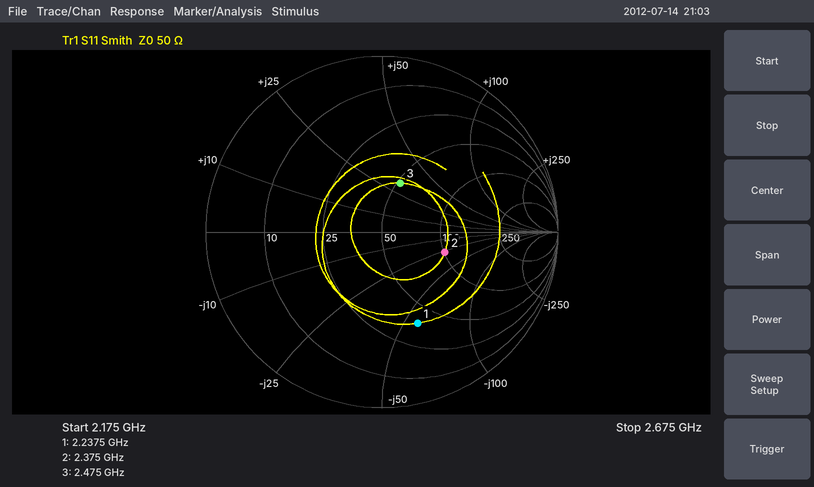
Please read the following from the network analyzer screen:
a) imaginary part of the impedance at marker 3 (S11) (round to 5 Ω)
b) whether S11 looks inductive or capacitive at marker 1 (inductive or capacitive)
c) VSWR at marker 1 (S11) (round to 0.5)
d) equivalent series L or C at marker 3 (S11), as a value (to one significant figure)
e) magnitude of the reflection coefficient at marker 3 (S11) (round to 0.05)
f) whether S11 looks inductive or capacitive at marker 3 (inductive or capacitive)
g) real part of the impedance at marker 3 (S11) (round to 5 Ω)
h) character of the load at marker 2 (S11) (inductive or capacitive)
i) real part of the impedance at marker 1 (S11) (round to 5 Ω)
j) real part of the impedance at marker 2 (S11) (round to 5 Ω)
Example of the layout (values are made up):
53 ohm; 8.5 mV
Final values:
+30 Ω; capacitive; 3.5; 2 nH; 0.30; inductive; 50 Ω; capacitive; 40 Ω; 100 Ω
